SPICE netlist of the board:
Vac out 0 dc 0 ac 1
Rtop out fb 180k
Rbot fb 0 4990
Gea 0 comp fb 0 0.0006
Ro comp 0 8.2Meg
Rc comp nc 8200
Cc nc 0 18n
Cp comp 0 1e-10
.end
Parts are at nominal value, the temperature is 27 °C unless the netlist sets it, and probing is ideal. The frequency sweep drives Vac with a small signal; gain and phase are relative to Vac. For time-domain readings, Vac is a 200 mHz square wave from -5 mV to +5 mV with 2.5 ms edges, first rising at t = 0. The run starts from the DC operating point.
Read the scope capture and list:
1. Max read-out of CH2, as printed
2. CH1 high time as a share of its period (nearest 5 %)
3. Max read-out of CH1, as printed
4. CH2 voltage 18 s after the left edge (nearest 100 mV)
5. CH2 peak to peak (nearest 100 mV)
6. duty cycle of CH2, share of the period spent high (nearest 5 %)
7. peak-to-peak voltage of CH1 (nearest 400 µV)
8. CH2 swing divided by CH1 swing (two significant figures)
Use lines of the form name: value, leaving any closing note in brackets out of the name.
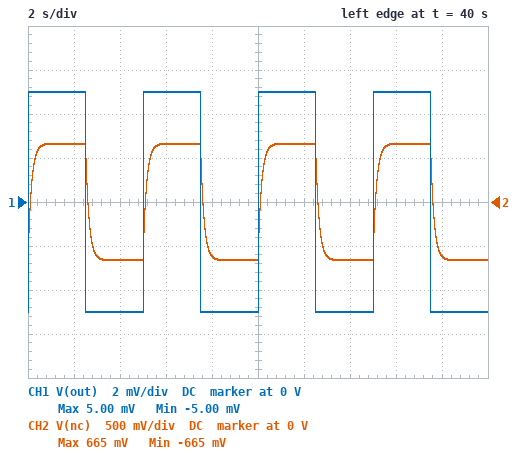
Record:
Max read-out of CH2, as printed: 665 mV
CH1 high time as a share of its period: 50 %
Max read-out of CH1, as printed: 5.00 mV
CH2 voltage 18 s after the left edge: -600 mV
CH2 peak to peak: 1.3 V
duty cycle of CH2, share of the period spent high: 50 %
peak-to-peak voltage of CH1: 10.0 mV
CH2 swing divided by CH1 swing: 130
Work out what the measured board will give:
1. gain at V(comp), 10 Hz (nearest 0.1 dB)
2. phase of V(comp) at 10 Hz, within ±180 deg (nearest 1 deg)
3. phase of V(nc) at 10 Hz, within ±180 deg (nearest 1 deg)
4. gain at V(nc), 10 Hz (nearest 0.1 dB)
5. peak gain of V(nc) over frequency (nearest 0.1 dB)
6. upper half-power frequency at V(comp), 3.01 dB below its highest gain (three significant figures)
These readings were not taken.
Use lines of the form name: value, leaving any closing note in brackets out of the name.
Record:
gain at V(comp), 10 Hz: 23.0 dB
phase of V(comp) at 10 Hz, within ±180 deg: -83 deg
phase of V(nc) at 10 Hz, within ±180 deg: -84 deg
gain at V(nc), 10 Hz: 23.0 dB
peak gain of V(nc) over frequency: 42.5 dB
upper half-power frequency at V(comp), 3.01 dB below its highest gain: 1.07 Hz
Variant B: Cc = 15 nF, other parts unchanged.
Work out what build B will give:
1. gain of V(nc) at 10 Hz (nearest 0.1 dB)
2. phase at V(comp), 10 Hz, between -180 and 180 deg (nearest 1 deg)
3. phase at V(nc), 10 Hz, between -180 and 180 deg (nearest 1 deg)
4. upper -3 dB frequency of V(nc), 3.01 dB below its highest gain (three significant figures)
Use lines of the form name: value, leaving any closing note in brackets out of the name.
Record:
gain of V(nc) at 10 Hz: 24.6 dB
phase at V(comp), 10 Hz, between -180 and 180 deg: -82 deg
phase at V(nc), 10 Hz, between -180 and 180 deg: -83 deg
upper -3 dB frequency of V(nc), 3.01 dB below its highest gain: 1.28 Hz
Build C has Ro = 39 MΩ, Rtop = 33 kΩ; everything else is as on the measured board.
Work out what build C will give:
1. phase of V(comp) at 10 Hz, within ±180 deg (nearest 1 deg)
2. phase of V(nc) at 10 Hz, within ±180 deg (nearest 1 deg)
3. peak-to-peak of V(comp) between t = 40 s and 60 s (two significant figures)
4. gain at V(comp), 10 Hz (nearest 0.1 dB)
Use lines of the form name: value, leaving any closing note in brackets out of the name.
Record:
phase of V(comp) at 10 Hz, within ±180 deg: -88 deg
phase of V(nc) at 10 Hz, within ±180 deg: -89 deg
peak-to-peak of V(comp) between t = 40 s and 60 s: 29 V
gain at V(comp), 10 Hz: 36.8 dB
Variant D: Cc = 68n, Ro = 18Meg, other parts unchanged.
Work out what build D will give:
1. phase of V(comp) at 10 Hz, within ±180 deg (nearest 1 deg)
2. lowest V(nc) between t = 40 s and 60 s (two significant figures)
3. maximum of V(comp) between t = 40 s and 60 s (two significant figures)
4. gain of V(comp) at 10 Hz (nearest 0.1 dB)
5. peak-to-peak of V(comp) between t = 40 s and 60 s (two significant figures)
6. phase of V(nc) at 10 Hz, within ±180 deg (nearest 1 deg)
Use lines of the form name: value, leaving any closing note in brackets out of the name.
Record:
phase of V(comp) at 10 Hz, within ±180 deg: -87 deg
lowest V(nc) between t = 40 s and 60 s: -1.1 V
maximum of V(comp) between t = 40 s and 60 s: 1.1 V
gain of V(comp) at 10 Hz: 11.6 dB
peak-to-peak of V(comp) between t = 40 s and 60 s: 2.2 V
phase of V(nc) at 10 Hz, within ±180 deg: -89 deg
